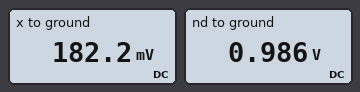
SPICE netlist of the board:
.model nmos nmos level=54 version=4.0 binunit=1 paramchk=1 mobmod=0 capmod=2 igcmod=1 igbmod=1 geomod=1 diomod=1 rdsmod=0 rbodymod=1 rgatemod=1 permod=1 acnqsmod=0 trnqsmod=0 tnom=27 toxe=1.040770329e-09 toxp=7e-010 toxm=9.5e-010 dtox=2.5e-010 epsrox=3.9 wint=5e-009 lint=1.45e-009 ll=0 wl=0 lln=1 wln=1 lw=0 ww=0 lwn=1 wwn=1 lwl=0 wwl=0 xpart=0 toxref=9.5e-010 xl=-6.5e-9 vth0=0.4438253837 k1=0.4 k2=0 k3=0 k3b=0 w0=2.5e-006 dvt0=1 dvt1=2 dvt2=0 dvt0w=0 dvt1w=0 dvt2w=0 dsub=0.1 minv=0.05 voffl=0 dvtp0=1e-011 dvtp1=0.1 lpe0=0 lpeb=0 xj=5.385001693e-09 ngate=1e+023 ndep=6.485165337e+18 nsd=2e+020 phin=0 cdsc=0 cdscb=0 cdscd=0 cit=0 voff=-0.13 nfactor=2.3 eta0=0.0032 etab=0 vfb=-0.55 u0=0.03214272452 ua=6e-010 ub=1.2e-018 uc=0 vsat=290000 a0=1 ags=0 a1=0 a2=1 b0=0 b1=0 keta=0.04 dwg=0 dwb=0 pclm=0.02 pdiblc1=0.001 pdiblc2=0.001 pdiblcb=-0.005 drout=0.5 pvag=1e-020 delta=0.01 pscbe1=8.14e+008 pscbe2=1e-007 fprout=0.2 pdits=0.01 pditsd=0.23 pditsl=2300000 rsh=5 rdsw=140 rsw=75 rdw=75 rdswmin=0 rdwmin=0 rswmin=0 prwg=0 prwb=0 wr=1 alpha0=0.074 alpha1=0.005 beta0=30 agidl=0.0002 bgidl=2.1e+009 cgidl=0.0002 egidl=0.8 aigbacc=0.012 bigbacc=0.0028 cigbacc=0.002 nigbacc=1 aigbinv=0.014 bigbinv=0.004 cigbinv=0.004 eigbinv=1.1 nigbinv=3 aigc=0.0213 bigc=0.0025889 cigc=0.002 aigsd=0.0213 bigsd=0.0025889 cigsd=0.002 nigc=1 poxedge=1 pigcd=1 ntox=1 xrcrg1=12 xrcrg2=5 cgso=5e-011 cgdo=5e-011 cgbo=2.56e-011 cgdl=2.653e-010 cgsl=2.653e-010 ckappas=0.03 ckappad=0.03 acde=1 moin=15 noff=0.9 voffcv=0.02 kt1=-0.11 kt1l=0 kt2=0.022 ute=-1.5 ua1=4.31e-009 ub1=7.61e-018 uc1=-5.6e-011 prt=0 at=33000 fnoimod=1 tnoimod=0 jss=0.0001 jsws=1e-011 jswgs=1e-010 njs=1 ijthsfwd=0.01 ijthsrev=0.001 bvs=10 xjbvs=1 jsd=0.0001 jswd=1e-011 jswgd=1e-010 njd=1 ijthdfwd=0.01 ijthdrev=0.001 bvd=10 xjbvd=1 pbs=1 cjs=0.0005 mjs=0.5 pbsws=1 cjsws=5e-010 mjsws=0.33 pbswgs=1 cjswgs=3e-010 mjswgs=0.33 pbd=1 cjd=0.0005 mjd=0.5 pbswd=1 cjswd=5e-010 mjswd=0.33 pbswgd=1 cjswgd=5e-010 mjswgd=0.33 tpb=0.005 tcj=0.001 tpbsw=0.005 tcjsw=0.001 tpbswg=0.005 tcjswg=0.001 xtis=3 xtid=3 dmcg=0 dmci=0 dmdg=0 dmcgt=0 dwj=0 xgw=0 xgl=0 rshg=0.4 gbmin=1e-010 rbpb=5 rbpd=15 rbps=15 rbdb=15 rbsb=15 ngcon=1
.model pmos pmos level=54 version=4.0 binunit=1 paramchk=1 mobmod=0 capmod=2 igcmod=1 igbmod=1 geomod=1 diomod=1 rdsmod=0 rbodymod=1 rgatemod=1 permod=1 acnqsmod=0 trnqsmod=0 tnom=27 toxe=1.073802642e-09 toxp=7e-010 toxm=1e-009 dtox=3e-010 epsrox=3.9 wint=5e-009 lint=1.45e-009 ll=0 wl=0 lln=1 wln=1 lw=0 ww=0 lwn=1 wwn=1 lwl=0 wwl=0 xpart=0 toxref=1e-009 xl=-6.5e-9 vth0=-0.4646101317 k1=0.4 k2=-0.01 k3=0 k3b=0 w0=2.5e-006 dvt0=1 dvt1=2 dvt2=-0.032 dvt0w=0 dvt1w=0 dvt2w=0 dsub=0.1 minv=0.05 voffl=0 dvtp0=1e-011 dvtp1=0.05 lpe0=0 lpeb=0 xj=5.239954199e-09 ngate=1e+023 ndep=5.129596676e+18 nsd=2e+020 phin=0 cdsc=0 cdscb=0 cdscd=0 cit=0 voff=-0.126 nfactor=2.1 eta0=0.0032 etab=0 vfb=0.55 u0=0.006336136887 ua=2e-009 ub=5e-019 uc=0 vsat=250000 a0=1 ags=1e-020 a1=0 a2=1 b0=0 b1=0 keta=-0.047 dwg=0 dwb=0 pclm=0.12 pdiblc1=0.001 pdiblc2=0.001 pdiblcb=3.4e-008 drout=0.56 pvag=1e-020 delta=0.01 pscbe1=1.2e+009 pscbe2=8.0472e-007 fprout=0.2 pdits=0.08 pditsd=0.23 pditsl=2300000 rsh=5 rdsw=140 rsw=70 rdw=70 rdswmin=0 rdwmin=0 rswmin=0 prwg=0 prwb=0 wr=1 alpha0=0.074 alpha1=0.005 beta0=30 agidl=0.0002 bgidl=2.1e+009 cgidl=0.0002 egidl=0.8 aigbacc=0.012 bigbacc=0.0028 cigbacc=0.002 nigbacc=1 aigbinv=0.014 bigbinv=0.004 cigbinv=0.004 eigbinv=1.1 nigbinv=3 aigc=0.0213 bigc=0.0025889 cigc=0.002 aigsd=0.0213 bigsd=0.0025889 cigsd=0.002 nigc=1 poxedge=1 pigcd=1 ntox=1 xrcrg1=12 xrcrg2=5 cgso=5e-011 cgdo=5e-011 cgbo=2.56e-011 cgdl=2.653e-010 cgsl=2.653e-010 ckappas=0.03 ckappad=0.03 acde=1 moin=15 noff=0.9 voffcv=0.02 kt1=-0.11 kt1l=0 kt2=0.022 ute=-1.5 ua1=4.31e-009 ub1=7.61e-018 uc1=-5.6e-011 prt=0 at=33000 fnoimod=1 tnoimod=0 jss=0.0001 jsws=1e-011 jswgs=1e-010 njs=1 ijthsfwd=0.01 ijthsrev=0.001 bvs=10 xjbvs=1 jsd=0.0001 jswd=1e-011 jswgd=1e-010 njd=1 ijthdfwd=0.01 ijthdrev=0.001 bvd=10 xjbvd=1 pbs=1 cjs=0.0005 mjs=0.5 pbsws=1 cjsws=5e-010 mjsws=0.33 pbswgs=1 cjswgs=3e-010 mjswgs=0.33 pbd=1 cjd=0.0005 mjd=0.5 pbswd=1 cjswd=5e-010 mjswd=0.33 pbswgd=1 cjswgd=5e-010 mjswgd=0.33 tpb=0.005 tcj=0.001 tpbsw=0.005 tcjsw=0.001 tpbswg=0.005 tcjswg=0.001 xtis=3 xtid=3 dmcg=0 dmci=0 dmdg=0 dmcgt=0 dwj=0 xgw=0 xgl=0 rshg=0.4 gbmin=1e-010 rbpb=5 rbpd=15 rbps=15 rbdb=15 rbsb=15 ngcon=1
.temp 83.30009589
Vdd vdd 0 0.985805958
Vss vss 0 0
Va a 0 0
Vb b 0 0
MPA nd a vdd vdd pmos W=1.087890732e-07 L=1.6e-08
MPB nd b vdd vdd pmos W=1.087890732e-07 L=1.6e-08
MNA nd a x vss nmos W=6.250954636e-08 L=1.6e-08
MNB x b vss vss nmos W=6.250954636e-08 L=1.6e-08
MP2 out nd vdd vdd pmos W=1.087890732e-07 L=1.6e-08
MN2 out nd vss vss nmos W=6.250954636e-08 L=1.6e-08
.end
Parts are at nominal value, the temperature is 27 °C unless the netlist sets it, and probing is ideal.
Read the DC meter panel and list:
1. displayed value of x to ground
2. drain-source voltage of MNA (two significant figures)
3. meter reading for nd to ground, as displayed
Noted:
182.2 mV
800 mV
0.986 V
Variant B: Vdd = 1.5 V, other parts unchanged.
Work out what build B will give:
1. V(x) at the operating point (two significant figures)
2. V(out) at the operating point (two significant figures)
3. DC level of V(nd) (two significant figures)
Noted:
290 mV
150 mV
1.5 V
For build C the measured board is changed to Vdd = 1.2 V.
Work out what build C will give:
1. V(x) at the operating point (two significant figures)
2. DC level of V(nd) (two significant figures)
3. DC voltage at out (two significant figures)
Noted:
230 mV
1.2 V
28 mV
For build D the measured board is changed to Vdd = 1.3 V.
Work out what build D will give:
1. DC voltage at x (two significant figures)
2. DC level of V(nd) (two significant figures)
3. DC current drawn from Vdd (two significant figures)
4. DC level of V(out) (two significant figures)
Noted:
250 mV
1.3 V
15 µA
57 mV
